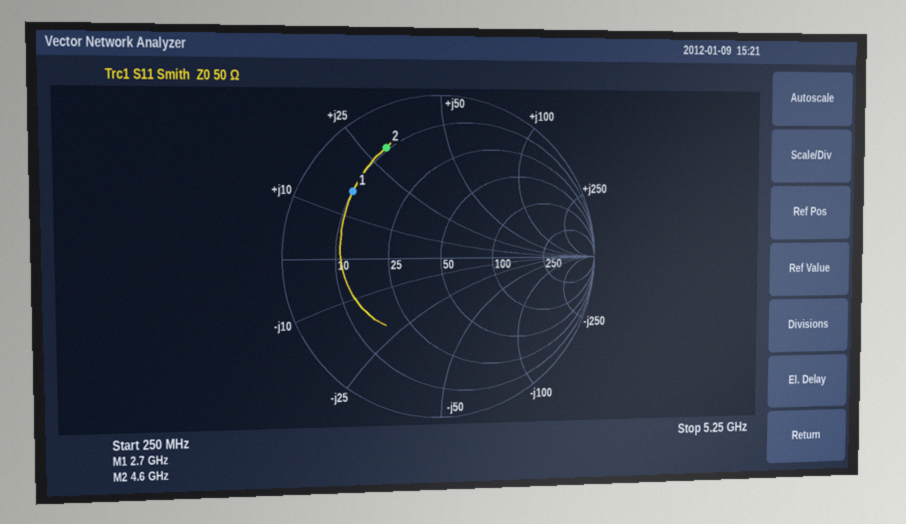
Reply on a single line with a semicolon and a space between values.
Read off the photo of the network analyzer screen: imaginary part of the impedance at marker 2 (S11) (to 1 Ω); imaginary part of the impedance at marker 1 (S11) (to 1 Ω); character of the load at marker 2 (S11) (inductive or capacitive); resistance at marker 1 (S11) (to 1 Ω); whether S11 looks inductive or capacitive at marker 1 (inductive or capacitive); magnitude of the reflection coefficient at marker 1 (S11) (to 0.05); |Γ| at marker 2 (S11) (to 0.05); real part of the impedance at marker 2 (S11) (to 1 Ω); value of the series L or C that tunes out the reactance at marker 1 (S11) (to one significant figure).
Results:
+30 Ω; +16 Ω; inductive; 10 Ω; inductive; 0.70; 0.75; 9 Ω; 4 pF
